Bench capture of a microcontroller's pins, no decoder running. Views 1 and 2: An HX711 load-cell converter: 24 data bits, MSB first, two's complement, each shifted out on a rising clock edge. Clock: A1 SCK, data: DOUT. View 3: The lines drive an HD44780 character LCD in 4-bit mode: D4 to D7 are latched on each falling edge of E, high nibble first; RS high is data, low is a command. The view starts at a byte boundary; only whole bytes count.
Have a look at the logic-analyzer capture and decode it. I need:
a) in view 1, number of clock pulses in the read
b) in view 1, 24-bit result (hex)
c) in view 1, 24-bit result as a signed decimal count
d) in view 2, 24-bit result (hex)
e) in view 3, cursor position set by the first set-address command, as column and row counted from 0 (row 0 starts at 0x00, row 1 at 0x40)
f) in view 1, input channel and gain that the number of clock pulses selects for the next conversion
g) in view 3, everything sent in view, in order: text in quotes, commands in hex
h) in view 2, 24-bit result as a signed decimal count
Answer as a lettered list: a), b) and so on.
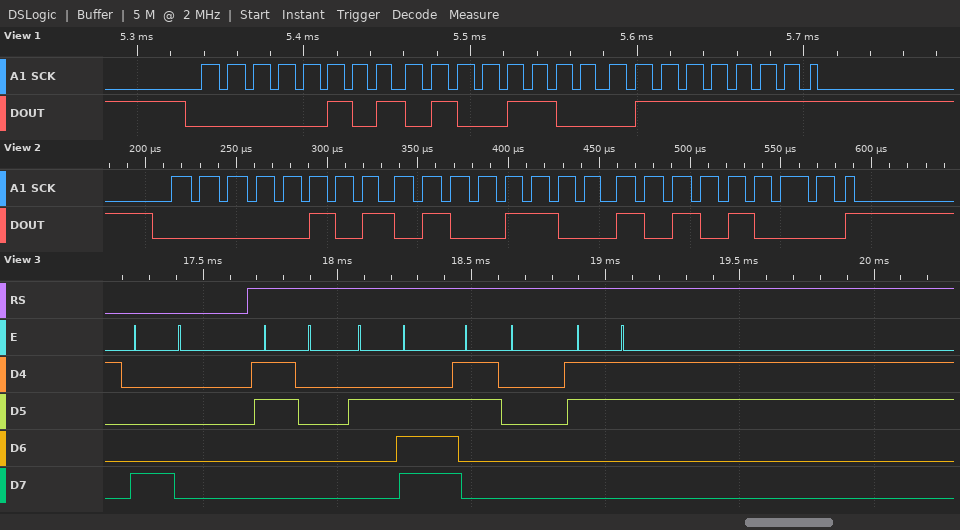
a) 25
b) 0x054C7F
c) 347263
d) 0x054CA8
e) column 0, row 0
f) channel A, gain 128
g) 0x80 "0.03"
h) 347304
